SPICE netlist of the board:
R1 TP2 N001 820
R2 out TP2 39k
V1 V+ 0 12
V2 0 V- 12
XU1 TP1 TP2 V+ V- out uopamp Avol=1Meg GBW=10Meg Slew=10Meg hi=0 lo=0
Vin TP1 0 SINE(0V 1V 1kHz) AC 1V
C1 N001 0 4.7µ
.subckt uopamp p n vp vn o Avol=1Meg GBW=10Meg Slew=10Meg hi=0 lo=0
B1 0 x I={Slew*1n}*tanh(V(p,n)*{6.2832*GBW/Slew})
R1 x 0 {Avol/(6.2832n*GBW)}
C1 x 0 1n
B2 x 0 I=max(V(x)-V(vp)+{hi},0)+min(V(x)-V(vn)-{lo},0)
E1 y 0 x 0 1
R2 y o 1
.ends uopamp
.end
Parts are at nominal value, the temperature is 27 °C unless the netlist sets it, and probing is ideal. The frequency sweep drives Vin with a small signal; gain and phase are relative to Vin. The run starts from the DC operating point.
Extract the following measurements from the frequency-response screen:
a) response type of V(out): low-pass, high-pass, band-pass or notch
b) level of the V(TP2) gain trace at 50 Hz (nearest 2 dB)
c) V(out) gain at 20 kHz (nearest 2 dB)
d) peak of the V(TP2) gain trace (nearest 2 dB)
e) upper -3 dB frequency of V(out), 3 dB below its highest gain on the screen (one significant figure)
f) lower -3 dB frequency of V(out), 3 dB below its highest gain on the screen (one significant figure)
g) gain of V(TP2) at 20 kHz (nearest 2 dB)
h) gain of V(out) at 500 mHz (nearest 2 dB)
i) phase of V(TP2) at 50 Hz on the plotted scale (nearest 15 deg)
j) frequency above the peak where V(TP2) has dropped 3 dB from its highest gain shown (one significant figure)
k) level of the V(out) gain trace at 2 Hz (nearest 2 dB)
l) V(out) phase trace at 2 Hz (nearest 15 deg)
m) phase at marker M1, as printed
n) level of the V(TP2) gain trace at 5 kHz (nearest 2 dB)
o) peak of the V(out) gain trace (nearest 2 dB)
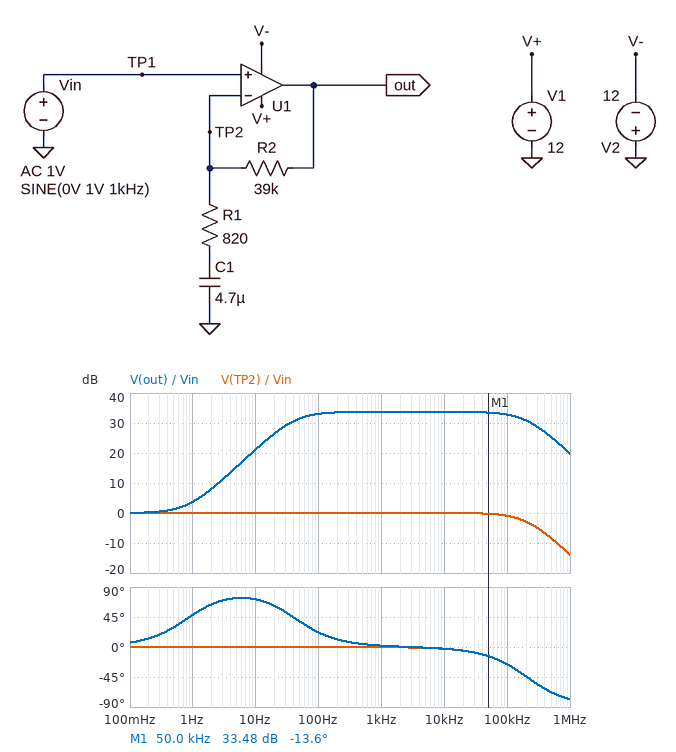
band-pass
0 dB
34 dB
0 dB
200 kHz
40 Hz
0 dB
2 dB
0 deg
200 kHz
8 dB
60 deg
-13.6 deg
0 dB
34 dB
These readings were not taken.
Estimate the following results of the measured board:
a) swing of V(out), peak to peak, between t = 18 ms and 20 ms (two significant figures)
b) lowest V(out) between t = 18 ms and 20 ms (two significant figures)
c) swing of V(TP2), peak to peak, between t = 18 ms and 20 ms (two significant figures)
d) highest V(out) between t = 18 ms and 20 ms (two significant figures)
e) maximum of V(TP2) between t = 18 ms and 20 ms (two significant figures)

24 V
-12 V
520 mV
12 V
270 mV
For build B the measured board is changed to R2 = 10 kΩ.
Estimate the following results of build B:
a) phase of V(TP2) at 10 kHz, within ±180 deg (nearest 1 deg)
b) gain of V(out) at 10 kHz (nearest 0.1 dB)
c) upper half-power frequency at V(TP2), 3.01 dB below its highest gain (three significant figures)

-1 deg
22.4 dB
758 kHz
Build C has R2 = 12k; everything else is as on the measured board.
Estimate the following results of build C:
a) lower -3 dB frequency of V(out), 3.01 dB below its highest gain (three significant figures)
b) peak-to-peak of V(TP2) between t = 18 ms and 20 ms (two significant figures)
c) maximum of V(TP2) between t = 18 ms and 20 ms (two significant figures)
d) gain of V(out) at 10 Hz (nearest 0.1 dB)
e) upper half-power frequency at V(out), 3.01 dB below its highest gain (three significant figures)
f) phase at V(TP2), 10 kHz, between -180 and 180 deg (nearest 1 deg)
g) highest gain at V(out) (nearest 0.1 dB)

41.1 Hz
1.6 V
790 mV
11.6 dB
640 kHz
-1 deg
23.9 dB
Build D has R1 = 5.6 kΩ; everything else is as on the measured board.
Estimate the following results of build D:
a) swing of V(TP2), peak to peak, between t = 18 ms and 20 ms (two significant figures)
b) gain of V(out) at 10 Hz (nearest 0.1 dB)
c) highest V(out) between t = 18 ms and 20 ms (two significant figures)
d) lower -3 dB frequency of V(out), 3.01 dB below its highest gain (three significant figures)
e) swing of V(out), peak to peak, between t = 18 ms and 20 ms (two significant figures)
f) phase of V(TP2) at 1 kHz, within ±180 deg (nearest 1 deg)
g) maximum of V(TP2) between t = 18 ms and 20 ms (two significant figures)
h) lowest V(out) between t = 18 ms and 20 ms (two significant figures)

2.0 V
16.7 dB
7.9 V
5.95 Hz
16 V
0 deg
1.0 V
-8.0 V
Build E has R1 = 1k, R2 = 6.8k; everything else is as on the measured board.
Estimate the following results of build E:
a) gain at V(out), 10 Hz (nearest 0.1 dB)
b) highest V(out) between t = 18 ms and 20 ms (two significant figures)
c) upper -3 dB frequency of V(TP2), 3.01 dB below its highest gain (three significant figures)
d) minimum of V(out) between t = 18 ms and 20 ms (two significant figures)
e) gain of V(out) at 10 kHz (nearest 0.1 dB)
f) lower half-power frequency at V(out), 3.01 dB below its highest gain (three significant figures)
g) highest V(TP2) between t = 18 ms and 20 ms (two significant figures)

7.6 dB
7.8 V
1.28 MHz
-7.8 V
17.8 dB
33.3 Hz
1.0 V
